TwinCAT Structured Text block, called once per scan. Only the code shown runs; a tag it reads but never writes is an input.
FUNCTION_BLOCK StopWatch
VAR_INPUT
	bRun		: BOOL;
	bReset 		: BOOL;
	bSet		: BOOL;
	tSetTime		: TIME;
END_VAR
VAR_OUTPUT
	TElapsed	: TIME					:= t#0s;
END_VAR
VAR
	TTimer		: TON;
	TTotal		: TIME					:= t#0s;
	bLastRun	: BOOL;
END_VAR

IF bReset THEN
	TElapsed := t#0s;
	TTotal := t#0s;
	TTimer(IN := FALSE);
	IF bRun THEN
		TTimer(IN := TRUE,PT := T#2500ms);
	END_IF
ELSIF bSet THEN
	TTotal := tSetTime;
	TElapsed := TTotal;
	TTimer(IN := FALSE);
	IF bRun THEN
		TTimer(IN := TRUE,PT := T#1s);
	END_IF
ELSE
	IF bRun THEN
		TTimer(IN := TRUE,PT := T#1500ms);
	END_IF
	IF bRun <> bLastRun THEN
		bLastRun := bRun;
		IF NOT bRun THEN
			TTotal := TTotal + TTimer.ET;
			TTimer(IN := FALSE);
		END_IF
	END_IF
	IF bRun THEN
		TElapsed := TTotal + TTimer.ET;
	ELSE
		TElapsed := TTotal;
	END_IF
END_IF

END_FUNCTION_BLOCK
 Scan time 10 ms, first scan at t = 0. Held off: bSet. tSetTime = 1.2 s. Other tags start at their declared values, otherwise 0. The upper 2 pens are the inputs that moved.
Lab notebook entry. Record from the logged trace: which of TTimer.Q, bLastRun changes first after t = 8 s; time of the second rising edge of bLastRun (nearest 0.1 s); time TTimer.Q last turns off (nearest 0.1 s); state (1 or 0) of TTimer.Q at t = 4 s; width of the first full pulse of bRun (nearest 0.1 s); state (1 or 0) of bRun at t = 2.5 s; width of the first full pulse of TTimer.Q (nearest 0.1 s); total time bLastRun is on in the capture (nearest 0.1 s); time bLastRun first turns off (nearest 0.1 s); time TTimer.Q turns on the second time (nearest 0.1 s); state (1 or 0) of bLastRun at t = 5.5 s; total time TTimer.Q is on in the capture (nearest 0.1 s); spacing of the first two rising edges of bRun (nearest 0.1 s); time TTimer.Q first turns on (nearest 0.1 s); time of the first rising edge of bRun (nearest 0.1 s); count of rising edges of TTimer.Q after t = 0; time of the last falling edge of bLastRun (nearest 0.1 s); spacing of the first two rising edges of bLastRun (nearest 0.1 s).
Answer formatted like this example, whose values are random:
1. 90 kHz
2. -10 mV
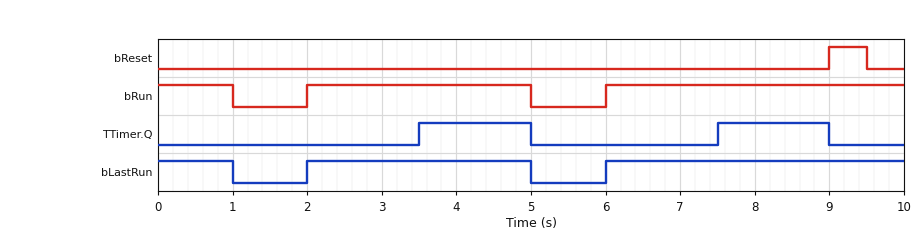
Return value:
1. TTimer.Q
2. 6.0 s
3. 9.0 s
4. 1
5. 3.0 s
6. 1
7. 1.5 s
8. 8.0 s
9. 1.0 s
10. 7.5 s
11. 0
12. 3.0 s
13. 4.0 s
14. 3.5 s
15. 2.0 s
16. 2
17. 5.0 s
18. 4.0 s
